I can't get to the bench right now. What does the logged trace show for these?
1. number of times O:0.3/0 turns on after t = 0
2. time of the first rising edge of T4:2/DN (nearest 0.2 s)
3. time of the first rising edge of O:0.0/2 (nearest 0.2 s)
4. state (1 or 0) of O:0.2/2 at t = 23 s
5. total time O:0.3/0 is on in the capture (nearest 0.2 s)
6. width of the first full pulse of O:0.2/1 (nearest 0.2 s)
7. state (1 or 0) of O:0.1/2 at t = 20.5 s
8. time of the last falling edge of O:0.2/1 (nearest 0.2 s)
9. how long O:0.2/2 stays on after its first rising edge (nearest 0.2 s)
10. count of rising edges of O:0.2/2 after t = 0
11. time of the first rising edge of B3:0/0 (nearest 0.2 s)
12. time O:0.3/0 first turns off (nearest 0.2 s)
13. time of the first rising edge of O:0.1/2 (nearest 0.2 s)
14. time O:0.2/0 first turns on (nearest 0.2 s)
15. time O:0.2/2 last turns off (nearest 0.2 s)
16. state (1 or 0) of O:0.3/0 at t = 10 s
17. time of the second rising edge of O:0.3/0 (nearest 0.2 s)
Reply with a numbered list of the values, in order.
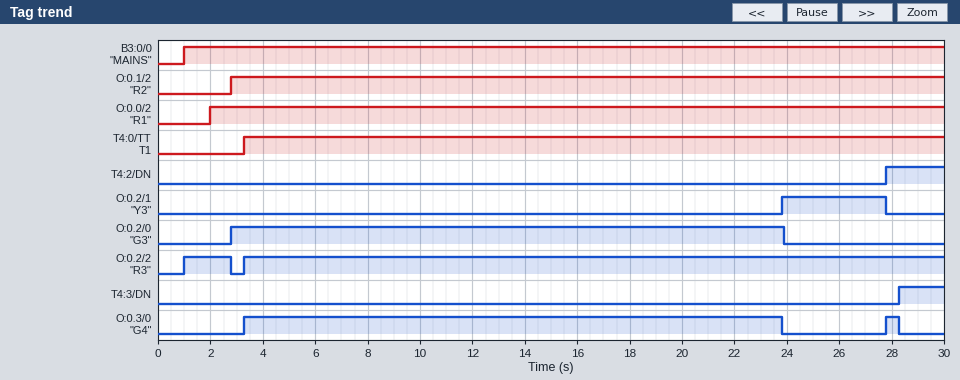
1. 2
2. 27.8 s
3. 2.0 s
4. 1
5. 21.0 s
6. 4.0 s
7. 1
8. 27.8 s
9. 1.8 s
10. 2
11. 1.0 s
12. 23.8 s
13. 2.8 s
14. 2.8 s
15. 2.8 s
16. 1
17. 27.8 s
